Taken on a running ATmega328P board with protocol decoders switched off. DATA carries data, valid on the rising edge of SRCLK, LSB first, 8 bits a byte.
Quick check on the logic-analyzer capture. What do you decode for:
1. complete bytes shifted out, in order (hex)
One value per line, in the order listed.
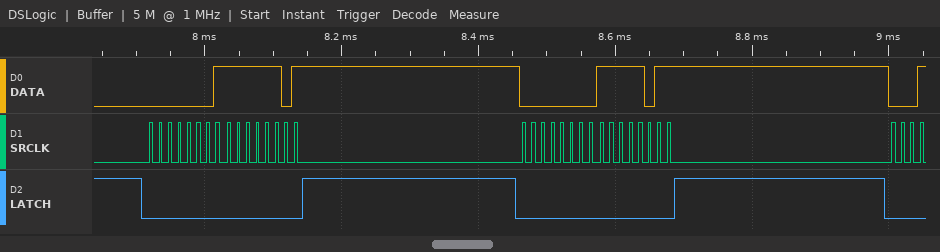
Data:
80 BF 00 DF
